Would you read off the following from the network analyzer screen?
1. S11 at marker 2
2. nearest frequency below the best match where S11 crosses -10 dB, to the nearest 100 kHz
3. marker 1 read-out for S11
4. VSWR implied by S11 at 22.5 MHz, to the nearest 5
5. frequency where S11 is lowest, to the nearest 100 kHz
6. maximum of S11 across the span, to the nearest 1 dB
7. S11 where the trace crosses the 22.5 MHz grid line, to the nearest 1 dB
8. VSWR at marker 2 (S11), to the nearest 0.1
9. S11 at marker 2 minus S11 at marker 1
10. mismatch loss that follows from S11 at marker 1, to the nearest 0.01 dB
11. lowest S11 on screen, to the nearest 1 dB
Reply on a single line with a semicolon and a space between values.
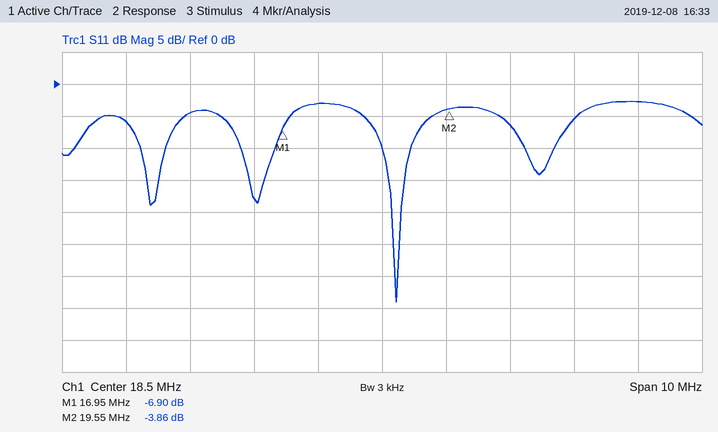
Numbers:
-3.86 dB; 18.5 MHz; -6.90 dB; 5; 18.7 MHz; -3 dB; -3 dB; 4.6; 3.04 dB; 0.99 dB; -34 dB
